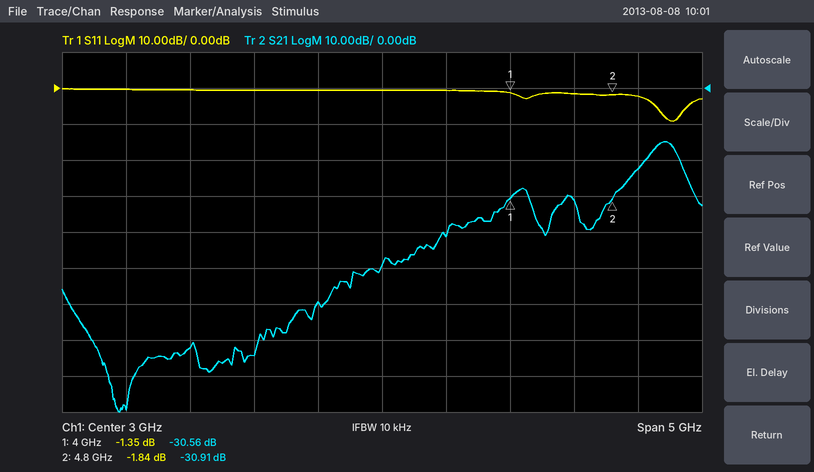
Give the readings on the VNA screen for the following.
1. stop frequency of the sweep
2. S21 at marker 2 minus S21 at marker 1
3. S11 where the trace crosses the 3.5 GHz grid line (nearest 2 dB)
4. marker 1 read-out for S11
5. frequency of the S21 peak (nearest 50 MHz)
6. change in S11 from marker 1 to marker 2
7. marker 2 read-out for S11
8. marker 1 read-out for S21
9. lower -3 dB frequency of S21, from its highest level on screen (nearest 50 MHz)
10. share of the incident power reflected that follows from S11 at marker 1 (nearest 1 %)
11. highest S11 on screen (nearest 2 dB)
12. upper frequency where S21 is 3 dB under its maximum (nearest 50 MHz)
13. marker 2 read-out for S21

5.5 GHz
-0.35 dB
0 dB
-1.35 dB
5.20 GHz
-0.49 dB
-1.84 dB
-30.56 dB
5.10 GHz
73 %
0 dB
5.30 GHz
-30.91 dB
